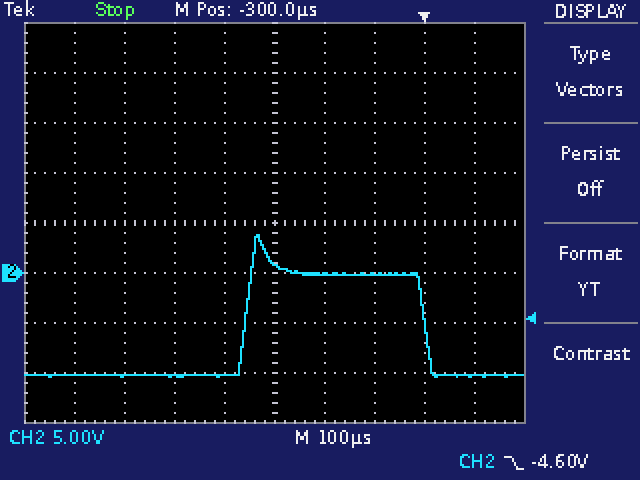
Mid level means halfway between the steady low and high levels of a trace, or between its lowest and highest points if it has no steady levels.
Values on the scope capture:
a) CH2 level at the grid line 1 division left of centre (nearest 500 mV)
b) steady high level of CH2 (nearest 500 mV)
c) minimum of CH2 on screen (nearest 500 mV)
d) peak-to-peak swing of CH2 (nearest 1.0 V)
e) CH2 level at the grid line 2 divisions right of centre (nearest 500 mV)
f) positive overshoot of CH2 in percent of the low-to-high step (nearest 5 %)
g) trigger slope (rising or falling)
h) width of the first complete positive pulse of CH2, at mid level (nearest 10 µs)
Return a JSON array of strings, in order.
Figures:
["-10.0 V", "0.0 V", "-10.5 V", "14.0 V", "0.0 V", "40 %", "falling", "360 µs"]
